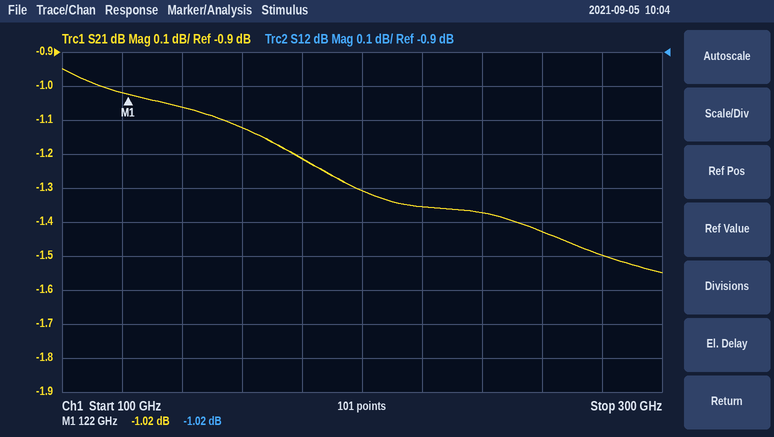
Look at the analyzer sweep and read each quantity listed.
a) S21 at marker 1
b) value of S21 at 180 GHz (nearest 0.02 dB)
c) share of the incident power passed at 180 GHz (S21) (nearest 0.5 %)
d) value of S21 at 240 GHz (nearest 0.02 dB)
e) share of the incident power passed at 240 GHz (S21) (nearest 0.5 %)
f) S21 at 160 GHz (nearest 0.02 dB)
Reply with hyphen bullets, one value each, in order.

- -1.02 dB
- -1.22 dB
- 75.5 %
- -1.38 dB
- 73.0 %
- -1.12 dB
